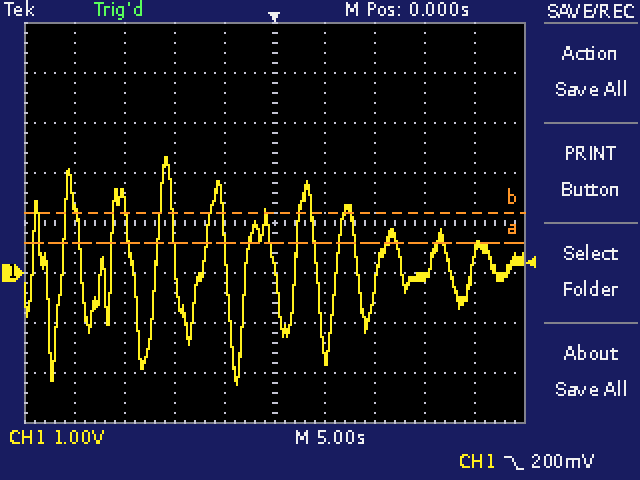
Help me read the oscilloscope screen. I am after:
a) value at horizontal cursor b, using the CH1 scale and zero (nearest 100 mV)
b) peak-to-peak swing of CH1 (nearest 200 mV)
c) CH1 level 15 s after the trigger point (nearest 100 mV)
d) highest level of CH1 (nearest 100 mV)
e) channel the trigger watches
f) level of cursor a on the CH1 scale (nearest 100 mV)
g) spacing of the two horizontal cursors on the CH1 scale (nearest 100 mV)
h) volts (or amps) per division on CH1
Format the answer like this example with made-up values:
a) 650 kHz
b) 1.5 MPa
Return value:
a) 1.2 V
b) 4.6 V
c) -100 mV
d) 2.3 V
e) CH1
f) 600 mV
g) 600 mV
h) 1 V
